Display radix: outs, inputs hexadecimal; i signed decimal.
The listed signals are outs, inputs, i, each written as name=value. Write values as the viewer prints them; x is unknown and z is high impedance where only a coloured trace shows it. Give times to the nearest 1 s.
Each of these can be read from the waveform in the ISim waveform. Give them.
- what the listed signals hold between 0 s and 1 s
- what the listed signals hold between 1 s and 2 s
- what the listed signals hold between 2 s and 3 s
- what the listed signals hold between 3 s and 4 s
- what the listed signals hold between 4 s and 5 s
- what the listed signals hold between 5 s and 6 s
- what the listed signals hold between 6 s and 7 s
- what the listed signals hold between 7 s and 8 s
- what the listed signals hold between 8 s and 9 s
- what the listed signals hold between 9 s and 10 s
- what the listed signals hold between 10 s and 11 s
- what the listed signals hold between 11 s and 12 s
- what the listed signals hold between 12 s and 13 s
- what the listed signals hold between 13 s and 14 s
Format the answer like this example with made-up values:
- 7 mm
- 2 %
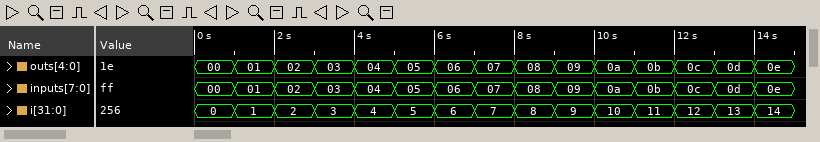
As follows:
- outs=00, inputs=00, i=0
- outs=01, inputs=01, i=1
- outs=02, inputs=02, i=2
- outs=03, inputs=03, i=3
- outs=04, inputs=04, i=4
- outs=05, inputs=05, i=5
- outs=06, inputs=06, i=6
- outs=07, inputs=07, i=7
- outs=08, inputs=08, i=8
- outs=09, inputs=09, i=9
- outs=0a, inputs=0a, i=10
- outs=0b, inputs=0b, i=11
- outs=0c, inputs=0c, i=12
- outs=0d, inputs=0d, i=13
